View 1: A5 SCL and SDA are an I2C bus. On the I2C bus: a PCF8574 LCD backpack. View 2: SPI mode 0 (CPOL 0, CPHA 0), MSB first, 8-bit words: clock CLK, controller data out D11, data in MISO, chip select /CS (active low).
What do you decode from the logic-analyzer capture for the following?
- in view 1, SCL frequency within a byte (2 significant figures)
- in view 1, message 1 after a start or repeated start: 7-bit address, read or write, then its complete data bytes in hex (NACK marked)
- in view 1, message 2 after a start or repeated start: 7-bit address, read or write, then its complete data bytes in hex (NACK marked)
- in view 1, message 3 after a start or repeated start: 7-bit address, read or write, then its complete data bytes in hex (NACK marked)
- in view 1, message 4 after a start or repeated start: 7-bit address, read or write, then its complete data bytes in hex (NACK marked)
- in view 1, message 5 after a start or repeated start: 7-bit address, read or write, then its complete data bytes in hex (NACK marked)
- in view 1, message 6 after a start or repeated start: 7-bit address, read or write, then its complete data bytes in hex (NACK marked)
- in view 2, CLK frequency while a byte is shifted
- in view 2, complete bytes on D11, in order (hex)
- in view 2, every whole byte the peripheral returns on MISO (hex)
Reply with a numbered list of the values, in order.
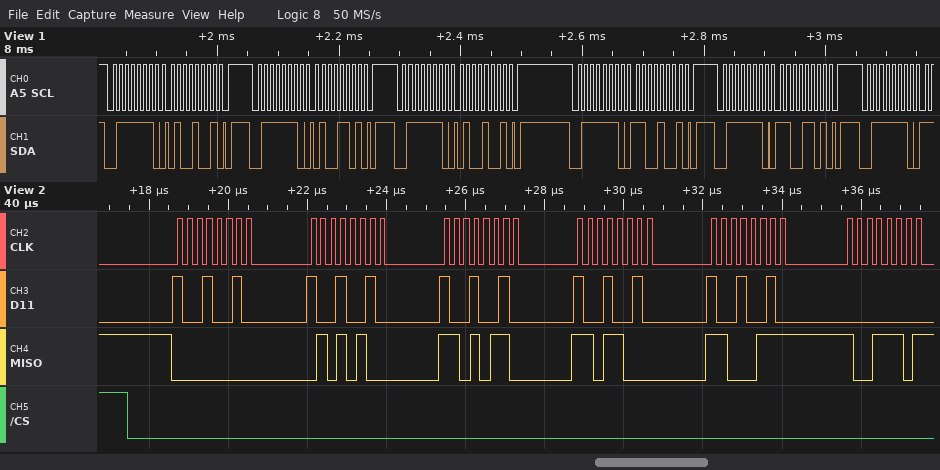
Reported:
1. 100 kHz
2. 0x3F write: 49
3. 0x3F write: 4D
4. 0x3F write: 49
5. 0x3F write: C9
6. 0x3F write: CD
7. 0x3F write
8. 4 MHz
9. 92 92 92 92 92 00
10. 00 54 D6 D8 C7 9D
